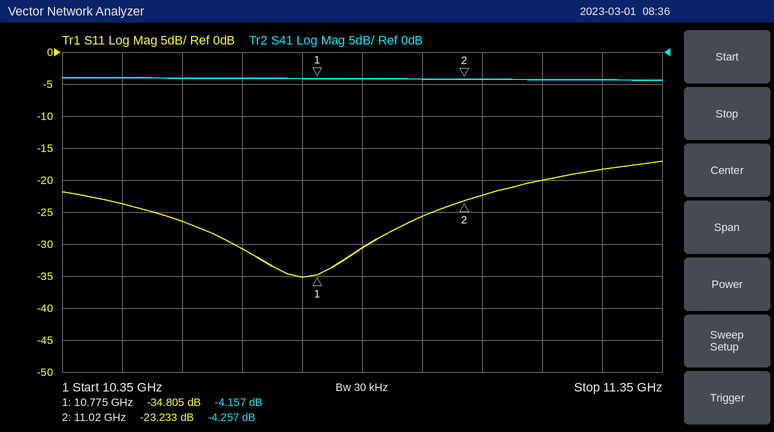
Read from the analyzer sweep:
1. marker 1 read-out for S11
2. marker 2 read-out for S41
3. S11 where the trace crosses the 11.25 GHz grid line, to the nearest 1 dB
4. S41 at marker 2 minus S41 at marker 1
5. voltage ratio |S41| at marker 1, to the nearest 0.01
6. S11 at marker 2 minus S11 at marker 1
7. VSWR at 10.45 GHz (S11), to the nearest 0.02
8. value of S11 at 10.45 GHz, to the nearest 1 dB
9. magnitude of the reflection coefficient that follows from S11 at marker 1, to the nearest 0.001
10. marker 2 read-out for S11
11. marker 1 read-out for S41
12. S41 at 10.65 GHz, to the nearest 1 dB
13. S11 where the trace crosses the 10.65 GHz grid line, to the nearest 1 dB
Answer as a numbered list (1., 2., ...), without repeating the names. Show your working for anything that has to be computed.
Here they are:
1. -34.805 dB
2. -4.257 dB
3. -18 dB
4. -4.257 − (-4.157) = -0.100 dB
5. 10^(-4.157/20) ≈ 0.62
6. -23.233 − (-34.805) = 11.572 dB
7. |Γ| = 10^(-24/20) = 0.0631; VSWR = (1 + 0.0631)/(1 − 0.0631) ≈ 1.13, so 1.14 to the nearest 0.02
8. -24 dB
9. 10^(-34.805/20) ≈ 0.018
10. -23.233 dB
11. -4.157 dB
12. -4 dB
13. -31 dB
